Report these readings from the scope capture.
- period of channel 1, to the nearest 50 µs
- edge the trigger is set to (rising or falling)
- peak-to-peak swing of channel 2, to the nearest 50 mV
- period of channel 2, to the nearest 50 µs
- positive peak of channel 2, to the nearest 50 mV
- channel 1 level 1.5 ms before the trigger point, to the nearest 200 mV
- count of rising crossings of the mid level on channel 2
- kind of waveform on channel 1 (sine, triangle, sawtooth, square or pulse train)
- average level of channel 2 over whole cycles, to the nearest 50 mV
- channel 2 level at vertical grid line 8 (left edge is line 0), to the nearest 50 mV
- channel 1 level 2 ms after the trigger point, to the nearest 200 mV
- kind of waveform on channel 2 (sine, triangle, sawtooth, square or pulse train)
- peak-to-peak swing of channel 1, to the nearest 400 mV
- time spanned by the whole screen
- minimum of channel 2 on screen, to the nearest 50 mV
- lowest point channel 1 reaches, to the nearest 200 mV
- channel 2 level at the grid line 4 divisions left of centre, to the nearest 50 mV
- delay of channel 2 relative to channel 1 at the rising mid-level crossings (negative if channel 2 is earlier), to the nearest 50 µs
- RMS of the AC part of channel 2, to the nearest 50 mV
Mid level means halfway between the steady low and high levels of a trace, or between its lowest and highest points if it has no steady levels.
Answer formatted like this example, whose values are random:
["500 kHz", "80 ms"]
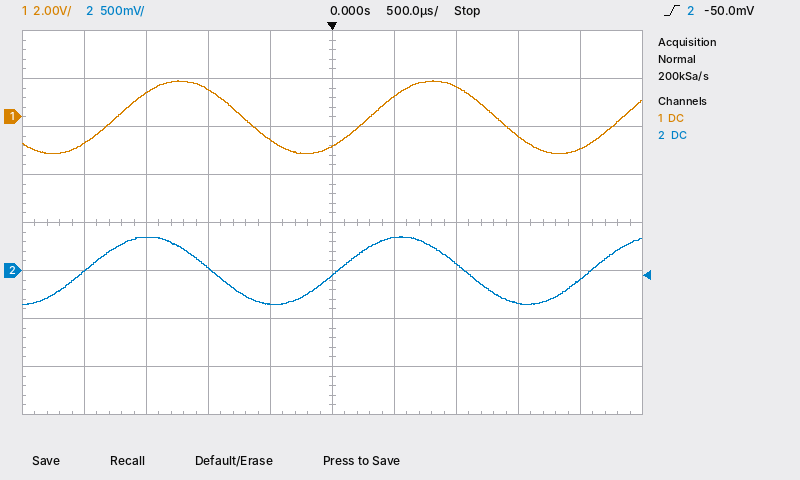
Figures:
["2.05 ms", "rising", "700 mV", "2.05 ms", "350 mV", "1.0 V", "3", "sine", "0 mV", "-350 mV", "-1.4 V", "sine", "3.2 V", "5 ms", "-350 mV", "-1.6 V", "0 mV", "-250 µs", "250 mV"]
